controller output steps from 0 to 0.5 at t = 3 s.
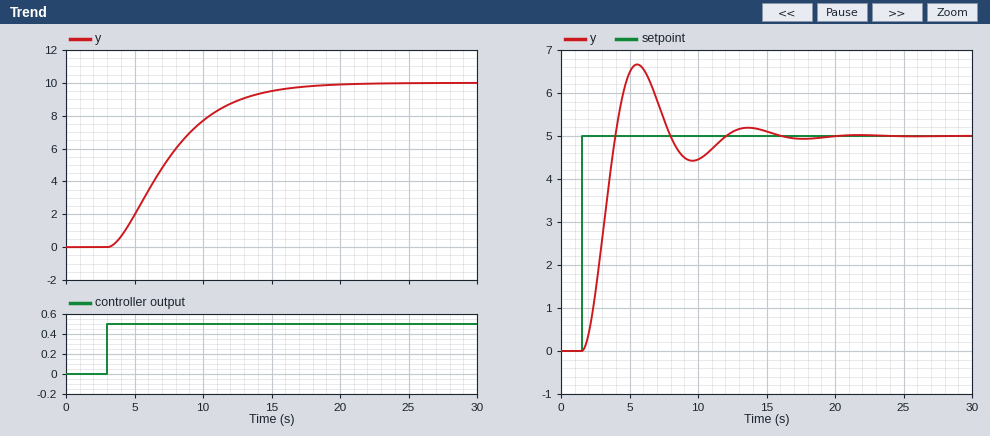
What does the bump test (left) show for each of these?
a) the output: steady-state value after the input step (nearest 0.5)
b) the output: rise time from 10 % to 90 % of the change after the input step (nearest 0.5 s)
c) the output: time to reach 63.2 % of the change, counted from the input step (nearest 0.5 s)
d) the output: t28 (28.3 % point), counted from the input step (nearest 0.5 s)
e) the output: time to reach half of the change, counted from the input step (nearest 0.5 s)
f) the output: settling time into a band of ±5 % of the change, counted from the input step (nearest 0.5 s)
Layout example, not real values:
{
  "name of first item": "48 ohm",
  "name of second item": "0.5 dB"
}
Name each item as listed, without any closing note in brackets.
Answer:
{
  "the output: steady-state value after the input step": "10.0",
  "the output: rise time from 10 % to 90 % of the change after the input step": "8.5 s",
  "the output: time to reach 63.2 % of the change, counted from the input step": "5.5 s",
  "the output: t28 (28.3 % point), counted from the input step": "2.5 s",
  "the output: time to reach half of the change, counted from the input step": "4.0 s",
  "the output: settling time into a band of ±5 % of the change, counted from the input step": "12.0 s"
}
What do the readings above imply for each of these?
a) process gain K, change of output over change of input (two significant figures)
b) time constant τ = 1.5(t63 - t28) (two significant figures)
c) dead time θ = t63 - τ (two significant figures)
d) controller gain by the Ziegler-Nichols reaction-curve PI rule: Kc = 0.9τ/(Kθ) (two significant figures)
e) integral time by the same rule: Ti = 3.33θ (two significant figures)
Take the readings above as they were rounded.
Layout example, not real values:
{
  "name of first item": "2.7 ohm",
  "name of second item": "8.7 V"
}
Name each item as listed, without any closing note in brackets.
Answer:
{
  "process gain K, change of output over change of input": "20",
  "time constant τ = 1.5(t63 - t28)": "4.5 s",
  "dead time θ = t63 - τ": "1.0 s",
  "controller gain by the Ziegler-Nichols reaction-curve PI rule: Kc = 0.9τ/(Kθ)": "0.20",
  "integral time by the same rule: Ti = 3.33θ": "3.3 s"
}
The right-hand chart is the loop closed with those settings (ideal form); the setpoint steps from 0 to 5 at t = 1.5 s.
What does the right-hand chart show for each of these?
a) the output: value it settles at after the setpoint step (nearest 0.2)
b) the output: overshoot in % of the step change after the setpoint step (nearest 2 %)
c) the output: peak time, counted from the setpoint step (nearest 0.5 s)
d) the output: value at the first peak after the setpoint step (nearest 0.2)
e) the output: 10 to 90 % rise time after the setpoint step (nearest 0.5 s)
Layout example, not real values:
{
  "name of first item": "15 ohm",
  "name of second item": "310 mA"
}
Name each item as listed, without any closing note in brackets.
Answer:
{
  "the output: value it settles at after the setpoint step": "5.0",
  "the output: overshoot in % of the step change after the setpoint step": "34 %",
  "the output: peak time, counted from the setpoint step": "4.0 s",
  "the output: value at the first peak after the setpoint step": "6.6",
  "the output: 10 to 90 % rise time after the setpoint step": "1.5 s"
}
